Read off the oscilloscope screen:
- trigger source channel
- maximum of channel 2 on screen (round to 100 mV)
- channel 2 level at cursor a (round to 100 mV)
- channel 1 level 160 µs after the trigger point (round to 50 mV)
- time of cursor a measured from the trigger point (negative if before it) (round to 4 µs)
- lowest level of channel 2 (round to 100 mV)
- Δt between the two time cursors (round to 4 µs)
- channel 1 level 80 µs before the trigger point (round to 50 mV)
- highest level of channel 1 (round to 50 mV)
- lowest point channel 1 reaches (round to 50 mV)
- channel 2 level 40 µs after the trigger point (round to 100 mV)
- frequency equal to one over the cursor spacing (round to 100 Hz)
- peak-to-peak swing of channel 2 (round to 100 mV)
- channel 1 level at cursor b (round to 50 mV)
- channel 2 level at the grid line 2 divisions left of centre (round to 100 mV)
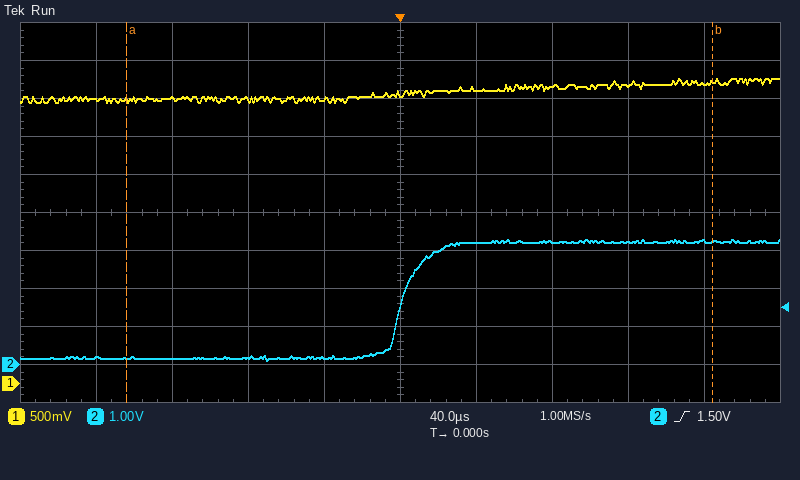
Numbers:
channel 2
3.3 V
200 mV
3.95 V
-144 µs
100 mV
308 µs
3.75 V
4.00 V
3.70 V
3.2 V
3.2 kHz
3.2 V
3.95 V
200 mV
